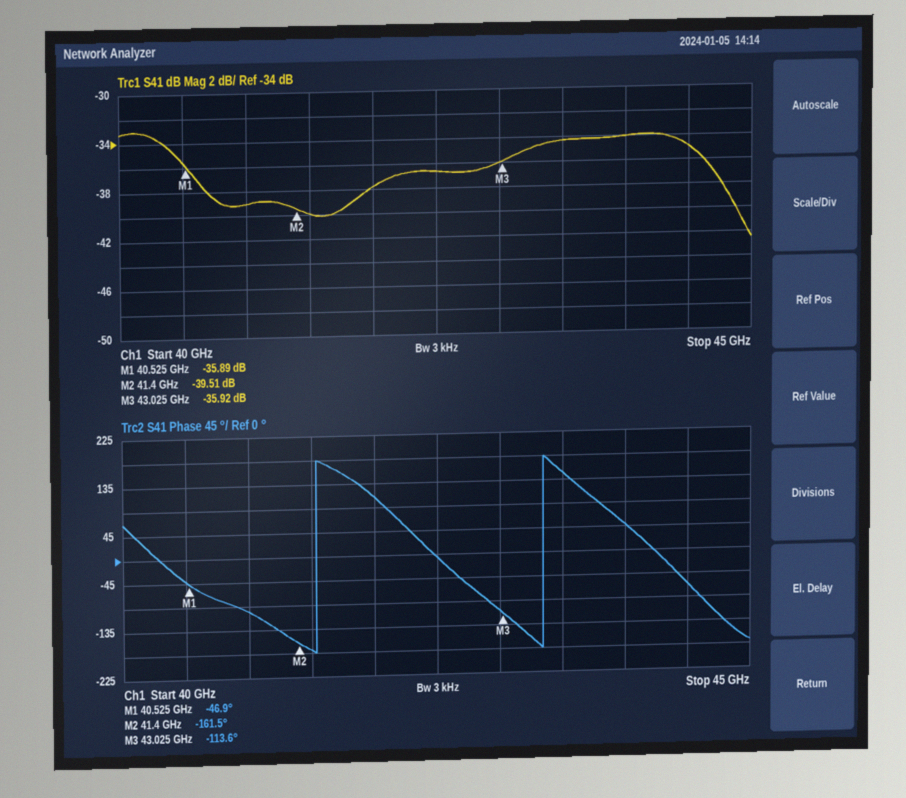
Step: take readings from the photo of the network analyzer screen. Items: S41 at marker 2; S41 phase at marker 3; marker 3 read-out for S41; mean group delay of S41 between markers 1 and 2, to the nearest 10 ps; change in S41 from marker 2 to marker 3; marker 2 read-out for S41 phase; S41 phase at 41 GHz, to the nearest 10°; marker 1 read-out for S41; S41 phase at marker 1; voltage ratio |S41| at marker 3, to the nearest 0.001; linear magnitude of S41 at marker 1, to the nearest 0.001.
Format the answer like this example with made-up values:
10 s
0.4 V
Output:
-39.51 dB
-113.6°
-35.92 dB
360 ps
3.59 dB
-161.5°
-100°
-35.89 dB
-46.9°
0.016
0.016
